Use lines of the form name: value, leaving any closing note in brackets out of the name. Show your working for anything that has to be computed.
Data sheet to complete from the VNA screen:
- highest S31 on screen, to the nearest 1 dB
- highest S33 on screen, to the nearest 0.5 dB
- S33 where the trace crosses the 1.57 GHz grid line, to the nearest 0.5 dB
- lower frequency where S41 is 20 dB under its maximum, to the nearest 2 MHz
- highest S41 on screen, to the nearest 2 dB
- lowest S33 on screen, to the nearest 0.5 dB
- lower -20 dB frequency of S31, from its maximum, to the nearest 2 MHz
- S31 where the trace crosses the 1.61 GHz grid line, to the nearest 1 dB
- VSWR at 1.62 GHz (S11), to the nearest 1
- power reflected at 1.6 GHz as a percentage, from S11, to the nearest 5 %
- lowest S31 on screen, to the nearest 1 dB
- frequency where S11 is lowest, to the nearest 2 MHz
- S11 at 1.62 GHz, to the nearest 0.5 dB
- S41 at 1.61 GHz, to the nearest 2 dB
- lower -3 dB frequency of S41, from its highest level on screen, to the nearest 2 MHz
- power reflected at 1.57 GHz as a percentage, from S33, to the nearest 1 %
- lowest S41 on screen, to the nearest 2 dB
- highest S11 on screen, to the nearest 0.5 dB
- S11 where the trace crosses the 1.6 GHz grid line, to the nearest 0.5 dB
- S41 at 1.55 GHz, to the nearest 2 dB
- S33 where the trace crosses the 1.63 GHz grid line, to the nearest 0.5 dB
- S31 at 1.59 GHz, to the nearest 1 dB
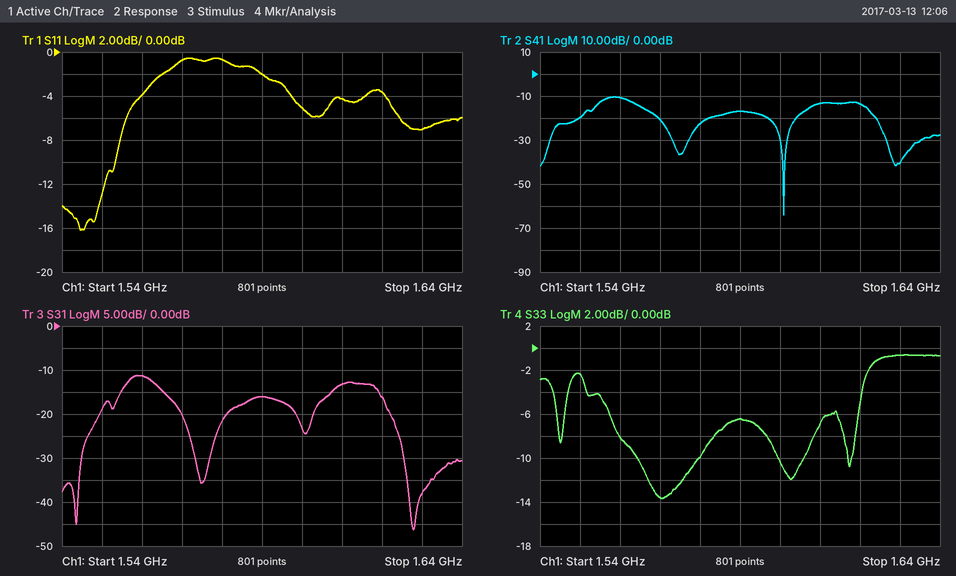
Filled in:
highest S31 on screen, to the nearest 1 dB: -11 dB
highest S33 on screen, to the nearest 0.5 dB: -0.5 dB
S33 where the trace crosses the 1.57 GHz grid line, to the nearest 0.5 dB: -13.5 dB
lower frequency where S41 is 20 dB under its maximum, to the nearest 2 MHz: 1.542 GHz
highest S41 on screen, to the nearest 2 dB: -10 dB
lowest S33 on screen, to the nearest 0.5 dB: -13.5 dB
lower -20 dB frequency of S31, from its maximum, to the nearest 2 MHz: 1.544 GHz
S31 where the trace crosses the 1.61 GHz grid line, to the nearest 1 dB: -13 dB
VSWR at 1.62 GHz (S11), to the nearest 1: |Γ| = 10^(-3.5/20) = 0.6683; VSWR = (1 + 0.6683)/(1 − 0.6683) ≈ 5
power reflected at 1.6 GHz as a percentage, from S11, to the nearest 5 %: 10^(-5/10) ≈ 31.6 %, so 30 % to the nearest 5 %
lowest S31 on screen, to the nearest 1 dB: -46 dB
frequency where S11 is lowest, to the nearest 2 MHz: 1.544 GHz
S11 at 1.62 GHz, to the nearest 0.5 dB: -3.5 dB
S41 at 1.61 GHz, to the nearest 2 dB: -14 dB
lower -3 dB frequency of S41, from its highest level on screen, to the nearest 2 MHz: 1.554 GHz
power reflected at 1.57 GHz as a percentage, from S33, to the nearest 1 %: 10^(-13.5/10) ≈ 4 %
lowest S41 on screen, to the nearest 2 dB: -64 dB
highest S11 on screen, to the nearest 0.5 dB: -0.5 dB
S11 where the trace crosses the 1.6 GHz grid line, to the nearest 0.5 dB: -5.0 dB
S41 at 1.55 GHz, to the nearest 2 dB: -20 dB
S33 where the trace crosses the 1.63 GHz grid line, to the nearest 0.5 dB: -0.5 dB
S31 at 1.59 GHz, to the nearest 1 dB: -16 dB
